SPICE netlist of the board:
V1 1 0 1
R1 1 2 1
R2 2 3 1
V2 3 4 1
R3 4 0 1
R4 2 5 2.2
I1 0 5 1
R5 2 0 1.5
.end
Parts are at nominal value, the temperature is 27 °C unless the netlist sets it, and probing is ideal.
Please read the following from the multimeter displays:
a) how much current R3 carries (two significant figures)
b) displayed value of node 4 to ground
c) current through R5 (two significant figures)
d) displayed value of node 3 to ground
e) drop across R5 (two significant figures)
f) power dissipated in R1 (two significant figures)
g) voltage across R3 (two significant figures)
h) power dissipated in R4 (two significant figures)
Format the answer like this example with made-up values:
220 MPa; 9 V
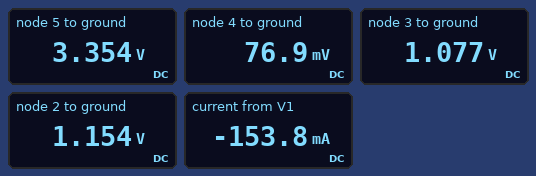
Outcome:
77 mA; 76.9 mV; 770 mA; 1.077 V; 1.2 V; 24 mW; 77 mV; 2.2 W
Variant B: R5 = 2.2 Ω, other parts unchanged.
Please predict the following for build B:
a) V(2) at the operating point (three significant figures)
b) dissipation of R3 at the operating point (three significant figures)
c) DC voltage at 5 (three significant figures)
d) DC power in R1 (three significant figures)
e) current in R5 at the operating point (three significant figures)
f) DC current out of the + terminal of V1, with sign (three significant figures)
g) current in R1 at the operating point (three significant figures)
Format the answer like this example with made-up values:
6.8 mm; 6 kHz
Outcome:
1.28 V; 19.5 mW; 3.48 V; 77.9 mW; 581 mA; -279 mA; 279 mA
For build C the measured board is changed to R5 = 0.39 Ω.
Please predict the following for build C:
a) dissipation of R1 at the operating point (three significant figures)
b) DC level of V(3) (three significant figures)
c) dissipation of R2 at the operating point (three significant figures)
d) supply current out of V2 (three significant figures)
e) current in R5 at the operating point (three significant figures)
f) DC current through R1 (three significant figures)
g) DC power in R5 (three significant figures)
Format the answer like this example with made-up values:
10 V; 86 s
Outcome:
148 mW; 808 mV; 37.0 mW; 192 mA; 1.58 A; 385 mA; 970 mW
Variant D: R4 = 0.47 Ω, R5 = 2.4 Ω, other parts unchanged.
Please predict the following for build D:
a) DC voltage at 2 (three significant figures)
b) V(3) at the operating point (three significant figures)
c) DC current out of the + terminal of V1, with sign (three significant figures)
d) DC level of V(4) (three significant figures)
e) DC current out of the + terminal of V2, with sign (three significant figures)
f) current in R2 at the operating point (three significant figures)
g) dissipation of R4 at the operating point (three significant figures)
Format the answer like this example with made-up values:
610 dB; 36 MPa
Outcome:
1.30 V; 1.15 V; -304 mA; 152 mV; -152 mA; 152 mA; 470 mW
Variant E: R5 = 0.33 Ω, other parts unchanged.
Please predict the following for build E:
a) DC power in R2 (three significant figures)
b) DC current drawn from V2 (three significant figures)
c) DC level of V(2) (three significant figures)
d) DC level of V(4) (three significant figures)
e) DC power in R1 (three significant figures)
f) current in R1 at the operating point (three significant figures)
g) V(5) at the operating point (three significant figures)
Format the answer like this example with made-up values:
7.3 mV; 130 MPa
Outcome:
50.2 mW; 224 mA; 552 mV; -224 mV; 201 mW; 448 mA; 2.75 V
